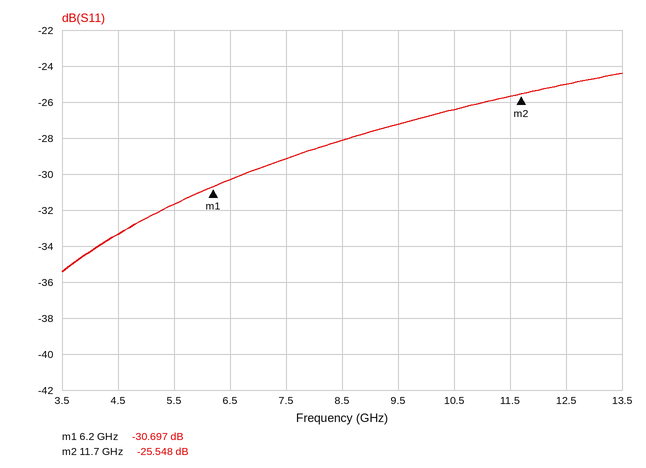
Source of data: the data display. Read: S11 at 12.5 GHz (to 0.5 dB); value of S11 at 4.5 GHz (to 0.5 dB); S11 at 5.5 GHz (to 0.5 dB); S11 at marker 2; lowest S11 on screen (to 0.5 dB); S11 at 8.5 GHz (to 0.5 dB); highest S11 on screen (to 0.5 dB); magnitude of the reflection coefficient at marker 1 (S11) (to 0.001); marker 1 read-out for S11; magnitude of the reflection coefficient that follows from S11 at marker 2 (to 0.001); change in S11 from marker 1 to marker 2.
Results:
-25.0 dB
-33.5 dB
-31.5 dB
-25.548 dB
-35.5 dB
-28.0 dB
-24.5 dB
0.029
-30.697 dB
0.053
5.149 dB
